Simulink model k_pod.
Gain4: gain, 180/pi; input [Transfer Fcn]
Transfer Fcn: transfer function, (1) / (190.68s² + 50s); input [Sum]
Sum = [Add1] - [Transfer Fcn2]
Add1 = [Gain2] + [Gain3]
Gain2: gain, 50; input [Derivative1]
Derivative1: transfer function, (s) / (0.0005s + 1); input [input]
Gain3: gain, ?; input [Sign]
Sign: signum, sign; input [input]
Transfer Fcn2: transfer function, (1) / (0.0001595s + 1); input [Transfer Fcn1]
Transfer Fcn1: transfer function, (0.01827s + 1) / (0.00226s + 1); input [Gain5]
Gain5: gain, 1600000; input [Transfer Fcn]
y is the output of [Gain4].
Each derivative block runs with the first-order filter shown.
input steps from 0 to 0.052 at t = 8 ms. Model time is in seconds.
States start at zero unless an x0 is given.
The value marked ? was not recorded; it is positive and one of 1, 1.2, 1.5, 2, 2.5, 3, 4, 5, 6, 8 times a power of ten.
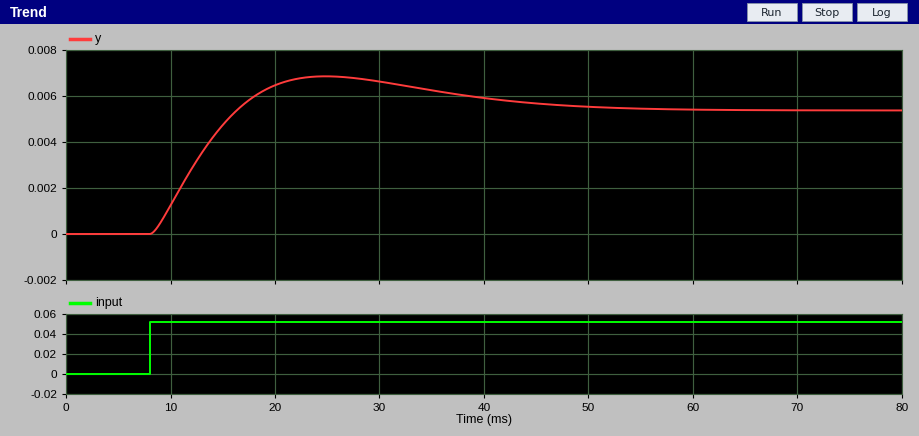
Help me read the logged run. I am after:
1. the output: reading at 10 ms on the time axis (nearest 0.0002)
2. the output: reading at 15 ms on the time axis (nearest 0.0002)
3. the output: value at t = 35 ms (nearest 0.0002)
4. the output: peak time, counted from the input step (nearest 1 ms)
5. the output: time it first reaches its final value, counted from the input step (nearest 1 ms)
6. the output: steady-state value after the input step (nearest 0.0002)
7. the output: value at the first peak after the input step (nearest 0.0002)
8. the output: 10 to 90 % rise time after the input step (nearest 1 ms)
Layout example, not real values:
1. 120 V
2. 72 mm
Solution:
1. 0.0012
2. 0.0048
3. 0.0062
4. 17 ms
5. 8 ms
6. 0.0054
7. 0.0068
8. 6 ms
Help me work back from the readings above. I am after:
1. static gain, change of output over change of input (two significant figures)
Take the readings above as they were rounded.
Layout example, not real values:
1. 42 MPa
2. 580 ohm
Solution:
1. 0.10
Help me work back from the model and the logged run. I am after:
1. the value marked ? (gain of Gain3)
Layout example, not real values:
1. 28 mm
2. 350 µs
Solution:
1. 150
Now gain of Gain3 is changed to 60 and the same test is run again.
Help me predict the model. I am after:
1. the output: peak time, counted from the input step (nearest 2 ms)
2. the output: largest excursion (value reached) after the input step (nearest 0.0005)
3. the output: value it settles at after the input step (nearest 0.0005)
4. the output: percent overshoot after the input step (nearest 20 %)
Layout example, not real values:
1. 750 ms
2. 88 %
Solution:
1. 12 ms
2. 0.0050
3. 0.0020
4. 140 %
